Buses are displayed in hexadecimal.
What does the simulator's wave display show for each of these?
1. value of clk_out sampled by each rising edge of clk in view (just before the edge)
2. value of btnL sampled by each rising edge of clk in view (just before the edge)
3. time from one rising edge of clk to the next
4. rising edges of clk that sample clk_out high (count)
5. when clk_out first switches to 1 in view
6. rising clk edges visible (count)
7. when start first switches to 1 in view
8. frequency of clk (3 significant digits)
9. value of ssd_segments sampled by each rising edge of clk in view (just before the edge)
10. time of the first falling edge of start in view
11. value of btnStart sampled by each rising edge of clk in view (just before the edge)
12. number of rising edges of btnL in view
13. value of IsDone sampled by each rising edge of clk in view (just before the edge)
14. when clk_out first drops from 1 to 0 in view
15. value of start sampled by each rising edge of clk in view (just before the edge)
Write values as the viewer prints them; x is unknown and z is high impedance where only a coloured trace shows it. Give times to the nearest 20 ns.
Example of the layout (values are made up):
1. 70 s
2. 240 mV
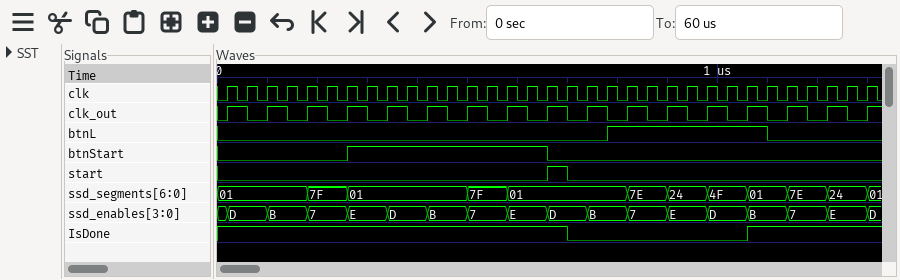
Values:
1. 0 1 0 1 0 1 0 1 0 1 0 1 0 1 0 1 0 1 0 1 0 1 0 1 0 1 0 1 0 1 0 1 0
2. 0 0 0 0 0 0 0 0 0 0 0 0 0 0 0 0 0 0 0 0 1 1 1 1 1 1 1 1 0 0 0 0 0
3. 40 ns
4. 16
5. 20 ns
6. 33
7. 660 ns
8. 25.0 MHz
9. 01, 01, 01, 01, 01, 7F, 7F, 01, 01, 01, 01, 01, 01, 7F, 7F, 01, 01, 01, 01, 01, 01, 7E, 7E, 24, 24, 4F, 4F, 01, 01, 7E, 7E, 24, 24
10. 700 ns
11. 0 0 0 0 0 0 0 1 1 1 1 1 1 1 1 1 1 0 0 0 0 0 0 0 0 0 0 0 0 0 0 0 0
12. 1
13. 1 1 1 1 1 1 1 1 1 1 1 1 1 1 1 1 1 1 0 0 0 0 0 0 0 0 0 1 1 1 1 1 1
14. 60 ns
15. 0 0 0 0 0 0 0 0 0 0 0 0 0 0 0 0 0 1 0 0 0 0 0 0 0 0 0 0 0 0 0 0 0
